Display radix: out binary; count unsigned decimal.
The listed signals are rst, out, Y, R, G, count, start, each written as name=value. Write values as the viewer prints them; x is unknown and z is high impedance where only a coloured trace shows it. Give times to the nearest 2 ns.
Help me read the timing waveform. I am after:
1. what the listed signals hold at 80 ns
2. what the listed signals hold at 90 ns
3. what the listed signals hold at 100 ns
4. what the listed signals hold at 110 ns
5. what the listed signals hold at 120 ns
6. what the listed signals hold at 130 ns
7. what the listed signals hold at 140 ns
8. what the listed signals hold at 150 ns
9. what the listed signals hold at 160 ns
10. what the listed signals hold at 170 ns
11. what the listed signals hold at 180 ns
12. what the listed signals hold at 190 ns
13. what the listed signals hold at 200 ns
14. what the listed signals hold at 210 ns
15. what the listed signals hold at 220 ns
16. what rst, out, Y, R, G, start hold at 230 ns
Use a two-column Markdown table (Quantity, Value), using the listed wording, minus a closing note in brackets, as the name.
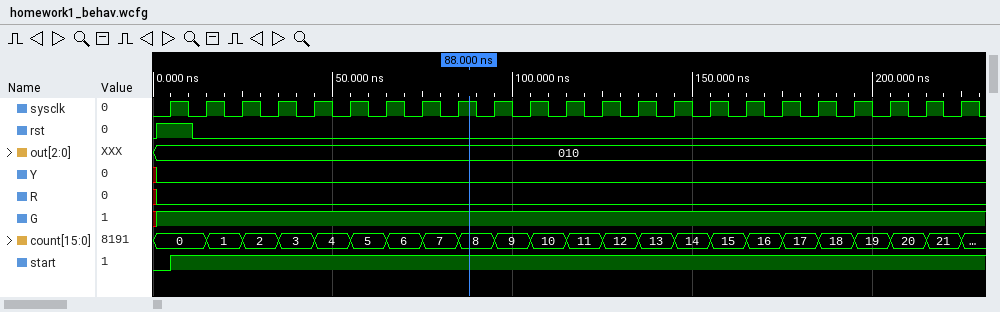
| Quantity | Value |
|---|---|
| what the listed signals hold at 80 ns | rst=0, out=010, Y=0, R=0, G=1, count=7, start=1 |
| what the listed signals hold at 90 ns | rst=0, out=010, Y=0, R=0, G=1, count=8, start=1 |
| what the listed signals hold at 100 ns | rst=0, out=010, Y=0, R=0, G=1, count=9, start=1 |
| what the listed signals hold at 110 ns | rst=0, out=010, Y=0, R=0, G=1, count=10, start=1 |
| what the listed signals hold at 120 ns | rst=0, out=010, Y=0, R=0, G=1, count=11, start=1 |
| what the listed signals hold at 130 ns | rst=0, out=010, Y=0, R=0, G=1, count=12, start=1 |
| what the listed signals hold at 140 ns | rst=0, out=010, Y=0, R=0, G=1, count=13, start=1 |
| what the listed signals hold at 150 ns | rst=0, out=010, Y=0, R=0, G=1, count=14, start=1 |
| what the listed signals hold at 160 ns | rst=0, out=010, Y=0, R=0, G=1, count=15, start=1 |
| what the listed signals hold at 170 ns | rst=0, out=010, Y=0, R=0, G=1, count=16, start=1 |
| what the listed signals hold at 180 ns | rst=0, out=010, Y=0, R=0, G=1, count=17, start=1 |
| what the listed signals hold at 190 ns | rst=0, out=010, Y=0, R=0, G=1, count=18, start=1 |
| what the listed signals hold at 200 ns | rst=0, out=010, Y=0, R=0, G=1, count=19, start=1 |
| what the listed signals hold at 210 ns | rst=0, out=010, Y=0, R=0, G=1, count=20, start=1 |
| what the listed signals hold at 220 ns | rst=0, out=010, Y=0, R=0, G=1, count=21, start=1 |
| what rst, out, Y, R, G, start hold at 230 ns | rst=0, out=010, Y=0, R=0, G=1, start=1 |
